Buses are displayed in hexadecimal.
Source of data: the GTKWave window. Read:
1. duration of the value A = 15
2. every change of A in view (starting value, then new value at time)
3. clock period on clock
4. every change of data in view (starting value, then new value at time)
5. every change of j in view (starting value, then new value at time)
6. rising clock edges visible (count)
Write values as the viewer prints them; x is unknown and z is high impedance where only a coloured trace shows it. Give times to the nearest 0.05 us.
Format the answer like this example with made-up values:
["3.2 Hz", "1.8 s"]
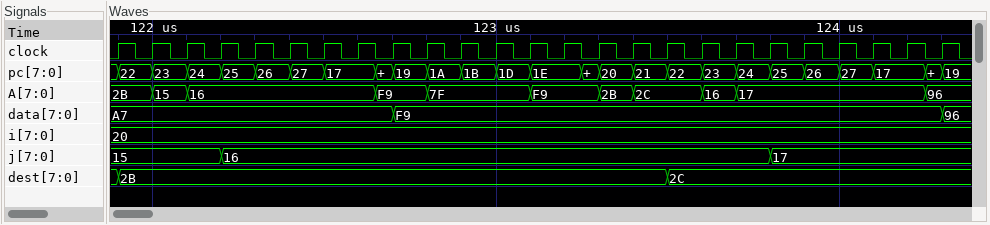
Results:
["0.1 us", "2B, 15 at 122 us, 16 at 122.1 us, F9 at 122.65 us, 7F at 122.8 us, F9 at 123.1 us, 2B at 123.3 us, 2C at 123.4 us, 16 at 123.6 us, 17 at 123.7 us, 96 at 124.25 us", "0.1 us", "A7, F9 at 122.7 us, 96 at 124.3 us", "15, 16 at 122.2 us, 17 at 123.8 us", "25"]
